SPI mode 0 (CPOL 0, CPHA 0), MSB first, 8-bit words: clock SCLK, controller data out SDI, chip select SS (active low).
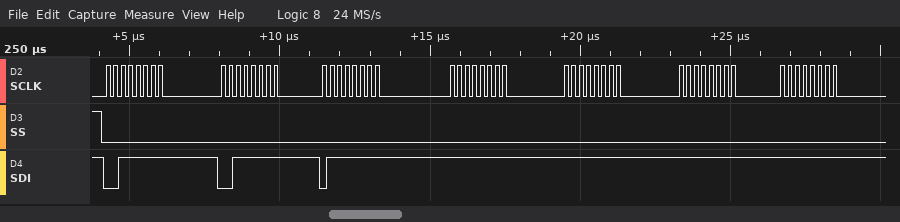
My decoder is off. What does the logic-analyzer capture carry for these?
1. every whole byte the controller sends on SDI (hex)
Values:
0x3F 0x3F 0x7F 0xFF 0xFF 0xFF 0xFF
